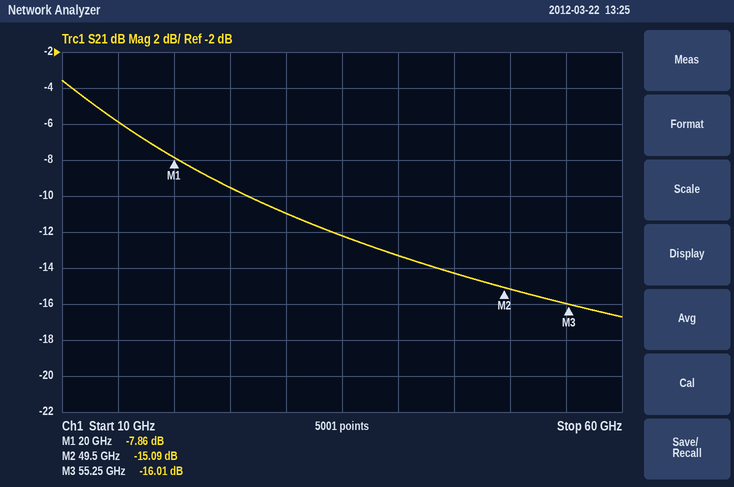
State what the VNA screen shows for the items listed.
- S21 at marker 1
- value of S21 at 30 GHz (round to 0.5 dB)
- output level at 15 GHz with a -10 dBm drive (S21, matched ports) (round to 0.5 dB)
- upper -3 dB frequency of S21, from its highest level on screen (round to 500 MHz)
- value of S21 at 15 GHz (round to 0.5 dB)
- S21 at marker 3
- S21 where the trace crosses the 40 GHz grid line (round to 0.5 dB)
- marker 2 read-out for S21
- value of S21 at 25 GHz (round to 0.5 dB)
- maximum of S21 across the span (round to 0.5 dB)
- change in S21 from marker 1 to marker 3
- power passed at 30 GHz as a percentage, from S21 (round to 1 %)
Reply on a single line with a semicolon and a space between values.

-7.86 dB; -11.0 dB; -16.0 dBm; 16.5 GHz; -6.0 dB; -16.01 dB; -13.5 dB; -15.09 dB; -9.5 dB; -3.5 dB; -8.15 dB; 8 %
